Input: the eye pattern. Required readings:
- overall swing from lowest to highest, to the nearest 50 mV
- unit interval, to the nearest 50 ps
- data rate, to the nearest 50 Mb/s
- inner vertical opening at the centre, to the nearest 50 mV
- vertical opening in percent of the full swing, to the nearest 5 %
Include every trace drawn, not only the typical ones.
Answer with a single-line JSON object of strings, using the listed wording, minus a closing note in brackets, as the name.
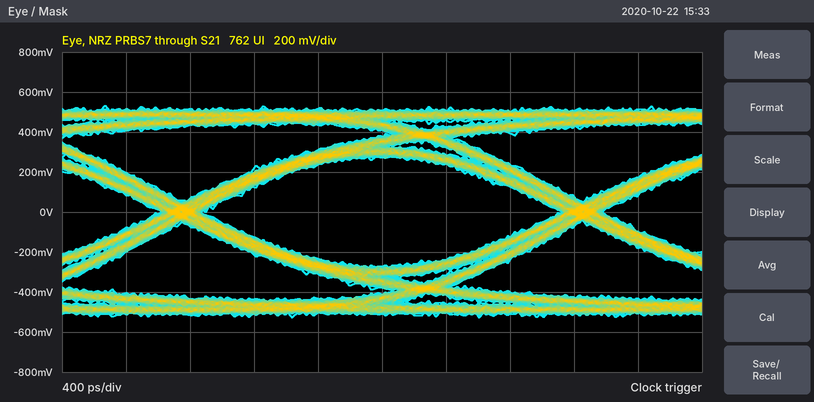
{"overall swing from lowest to highest, to the nearest 50 mV": "1.05 V", "unit interval, to the nearest 50 ps": "2.50 ns", "data rate, to the nearest 50 Mb/s": "400 Mb/s", "inner vertical opening at the centre, to the nearest 50 mV": "550 mV", "vertical opening in percent of the full swing, to the nearest 5 %": "50 %"}
